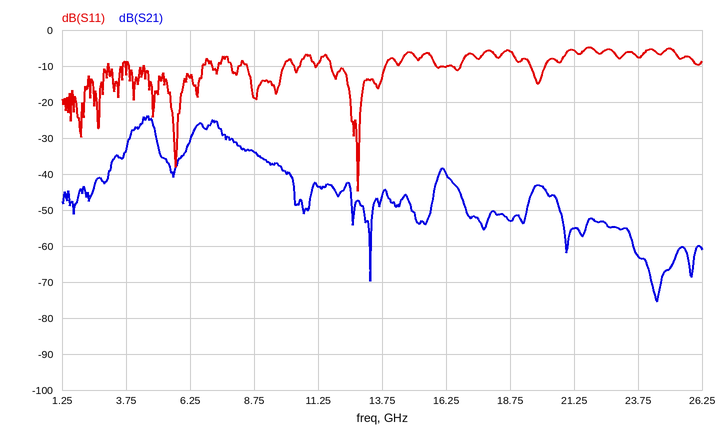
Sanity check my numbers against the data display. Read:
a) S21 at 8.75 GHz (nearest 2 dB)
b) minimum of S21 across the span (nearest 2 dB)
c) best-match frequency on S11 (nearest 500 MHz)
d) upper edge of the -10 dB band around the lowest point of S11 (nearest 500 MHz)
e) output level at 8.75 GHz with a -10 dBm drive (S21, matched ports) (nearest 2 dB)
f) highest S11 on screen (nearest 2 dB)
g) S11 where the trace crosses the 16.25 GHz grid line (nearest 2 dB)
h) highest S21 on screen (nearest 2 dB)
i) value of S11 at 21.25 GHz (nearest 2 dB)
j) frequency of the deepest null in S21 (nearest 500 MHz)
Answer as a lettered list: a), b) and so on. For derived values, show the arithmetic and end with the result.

a) -34 dB
b) -76 dB
c) 13.0 GHz
d) 14.0 GHz
e) -10 dBm + (-34 dB) = -44 dBm
f) -4 dB
g) -10 dB
h) -24 dB
i) -6 dB
j) 24.5 GHz
